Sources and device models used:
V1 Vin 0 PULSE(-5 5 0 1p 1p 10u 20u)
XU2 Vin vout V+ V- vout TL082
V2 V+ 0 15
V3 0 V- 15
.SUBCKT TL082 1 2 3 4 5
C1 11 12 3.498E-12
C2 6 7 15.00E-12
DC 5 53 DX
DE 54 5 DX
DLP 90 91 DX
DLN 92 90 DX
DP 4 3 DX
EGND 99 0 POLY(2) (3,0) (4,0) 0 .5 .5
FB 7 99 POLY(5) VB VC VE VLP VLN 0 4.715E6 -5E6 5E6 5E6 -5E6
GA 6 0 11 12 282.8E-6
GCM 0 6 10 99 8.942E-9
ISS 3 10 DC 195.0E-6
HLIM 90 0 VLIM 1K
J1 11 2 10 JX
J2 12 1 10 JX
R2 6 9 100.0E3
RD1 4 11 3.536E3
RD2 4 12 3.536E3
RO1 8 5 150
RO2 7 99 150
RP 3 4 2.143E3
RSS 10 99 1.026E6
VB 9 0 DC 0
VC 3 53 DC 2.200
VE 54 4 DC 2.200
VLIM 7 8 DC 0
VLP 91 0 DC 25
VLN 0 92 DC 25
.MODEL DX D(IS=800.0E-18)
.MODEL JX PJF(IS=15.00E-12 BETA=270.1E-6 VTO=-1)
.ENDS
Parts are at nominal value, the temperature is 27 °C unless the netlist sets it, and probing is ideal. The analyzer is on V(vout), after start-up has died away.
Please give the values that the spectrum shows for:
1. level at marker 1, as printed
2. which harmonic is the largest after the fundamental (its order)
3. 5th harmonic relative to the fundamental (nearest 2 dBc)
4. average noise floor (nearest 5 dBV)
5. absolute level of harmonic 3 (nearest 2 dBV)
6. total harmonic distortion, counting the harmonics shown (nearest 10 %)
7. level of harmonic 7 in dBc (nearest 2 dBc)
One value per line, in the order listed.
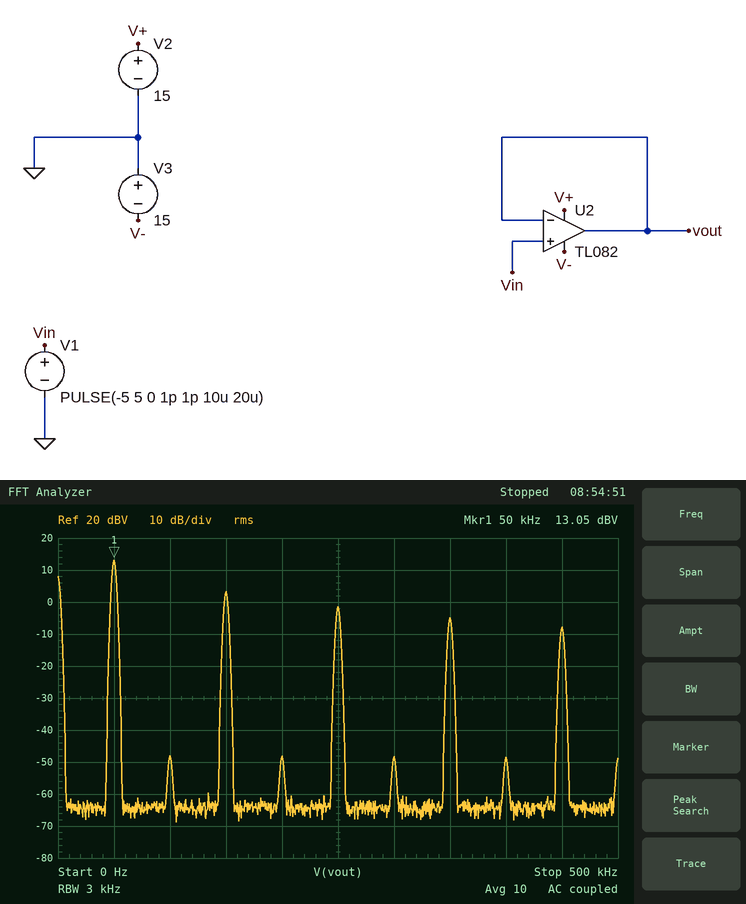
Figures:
13.05 dBV
3
-14 dBc
-65 dBV
4 dBV
40 %
-18 dBc
